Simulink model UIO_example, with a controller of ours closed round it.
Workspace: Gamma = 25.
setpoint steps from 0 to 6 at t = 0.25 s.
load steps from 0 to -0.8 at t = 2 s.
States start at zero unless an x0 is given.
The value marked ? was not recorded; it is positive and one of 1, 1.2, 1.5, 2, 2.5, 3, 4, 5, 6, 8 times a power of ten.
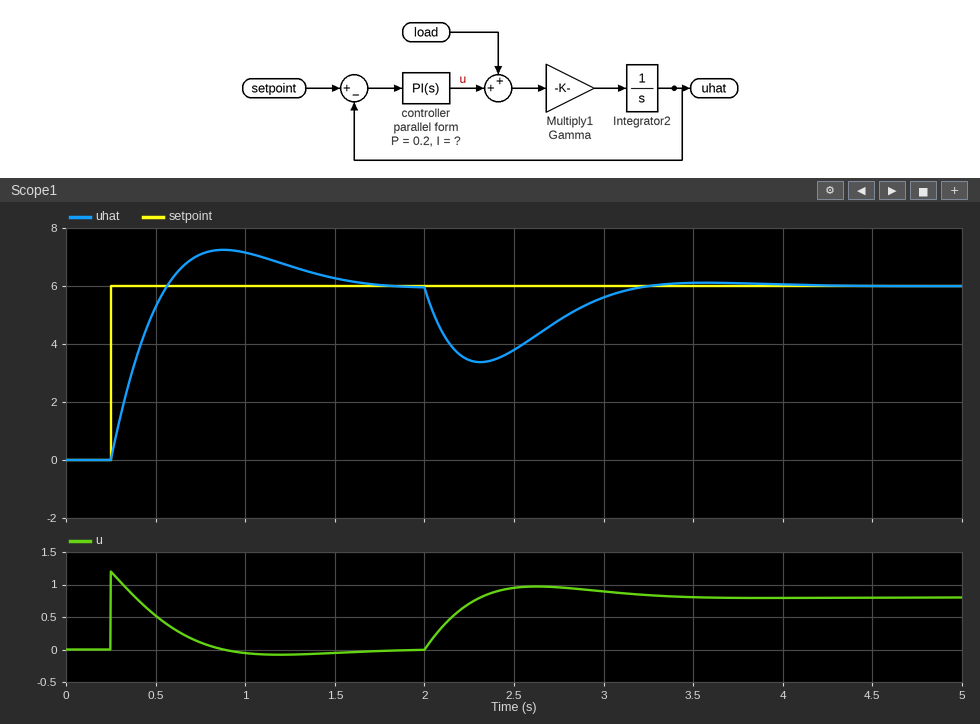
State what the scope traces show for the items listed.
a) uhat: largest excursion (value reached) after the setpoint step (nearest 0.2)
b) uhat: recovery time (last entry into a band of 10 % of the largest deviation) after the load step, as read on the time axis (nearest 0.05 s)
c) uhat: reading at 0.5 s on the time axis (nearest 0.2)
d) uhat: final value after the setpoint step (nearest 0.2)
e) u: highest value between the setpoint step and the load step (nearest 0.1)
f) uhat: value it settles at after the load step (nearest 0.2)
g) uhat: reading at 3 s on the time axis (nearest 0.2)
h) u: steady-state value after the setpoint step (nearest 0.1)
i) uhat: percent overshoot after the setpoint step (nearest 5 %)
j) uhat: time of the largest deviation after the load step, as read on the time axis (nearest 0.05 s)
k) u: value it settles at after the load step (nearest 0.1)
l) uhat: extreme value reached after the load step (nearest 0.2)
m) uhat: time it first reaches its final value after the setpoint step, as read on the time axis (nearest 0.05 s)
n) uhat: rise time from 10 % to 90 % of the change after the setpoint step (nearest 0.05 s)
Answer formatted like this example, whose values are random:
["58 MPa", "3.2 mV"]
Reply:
["7.2", "3.05 s", "5.2", "6.0", "1.2", "6.0", "5.6", "0.0", "20 %", "2.30 s", "0.8", "3.4", "0.55 s", "0.25 s"]
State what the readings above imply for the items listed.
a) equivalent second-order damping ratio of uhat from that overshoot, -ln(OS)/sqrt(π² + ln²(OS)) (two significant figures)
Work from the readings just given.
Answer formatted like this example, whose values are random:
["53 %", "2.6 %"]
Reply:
["0.46"]
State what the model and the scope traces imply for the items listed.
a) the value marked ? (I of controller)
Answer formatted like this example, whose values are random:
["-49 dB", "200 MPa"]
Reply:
["0.5"]
